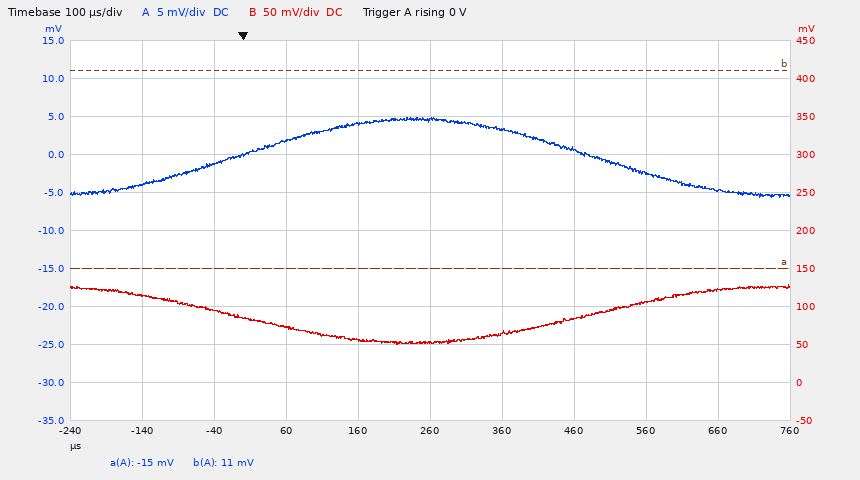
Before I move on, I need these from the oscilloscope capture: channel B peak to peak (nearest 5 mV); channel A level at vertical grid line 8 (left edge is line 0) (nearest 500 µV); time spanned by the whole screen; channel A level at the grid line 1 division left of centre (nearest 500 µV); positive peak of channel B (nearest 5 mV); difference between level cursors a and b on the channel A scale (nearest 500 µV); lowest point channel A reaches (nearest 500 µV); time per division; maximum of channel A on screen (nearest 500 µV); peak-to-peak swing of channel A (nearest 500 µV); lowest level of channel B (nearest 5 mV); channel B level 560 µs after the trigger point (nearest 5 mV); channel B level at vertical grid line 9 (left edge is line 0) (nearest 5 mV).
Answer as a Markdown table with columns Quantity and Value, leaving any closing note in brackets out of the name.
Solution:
| Quantity | Value |
|---|---|
| channel B peak to peak | 80 mV |
| channel A level at vertical grid line 8 (left edge is line 0) | -2.5 mV |
| time spanned by the whole screen | 1 ms |
| channel A level at the grid line 1 division left of centre | 4.0 mV |
| positive peak of channel B | 130 mV |
| difference between level cursors a and b on the channel A scale | 26.0 mV |
| lowest point channel A reaches | -5.5 mV |
| time per division | 100 µs |
| maximum of channel A on screen | 5.0 mV |
| peak-to-peak swing of channel A | 10.5 mV |
| lowest level of channel B | 50 mV |
| channel B level 560 µs after the trigger point | 105 mV |
| channel B level at vertical grid line 9 (left edge is line 0) | 120 mV |
